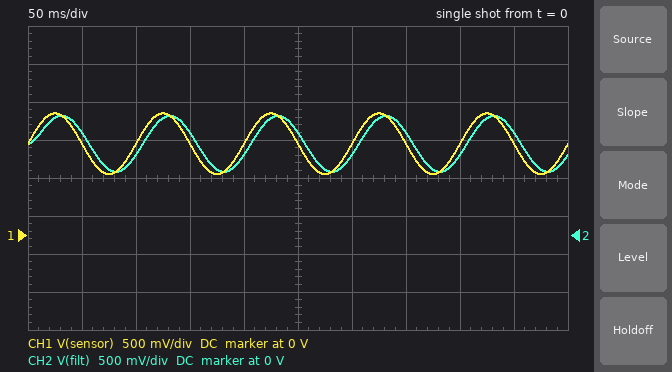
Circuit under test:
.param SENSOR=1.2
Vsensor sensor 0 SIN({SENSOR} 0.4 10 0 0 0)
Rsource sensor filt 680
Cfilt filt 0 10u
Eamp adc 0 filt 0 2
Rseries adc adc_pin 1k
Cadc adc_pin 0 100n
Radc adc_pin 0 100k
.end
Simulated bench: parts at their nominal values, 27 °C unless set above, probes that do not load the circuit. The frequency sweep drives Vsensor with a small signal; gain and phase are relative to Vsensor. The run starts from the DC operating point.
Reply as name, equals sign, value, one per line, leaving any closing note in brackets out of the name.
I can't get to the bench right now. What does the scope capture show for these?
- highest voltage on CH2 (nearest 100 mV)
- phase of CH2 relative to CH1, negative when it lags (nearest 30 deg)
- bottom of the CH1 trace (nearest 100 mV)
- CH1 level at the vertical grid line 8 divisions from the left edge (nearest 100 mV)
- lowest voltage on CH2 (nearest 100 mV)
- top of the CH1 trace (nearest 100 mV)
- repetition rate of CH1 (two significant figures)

highest voltage on CH2 = 1.6 V
phase of CH2 relative to CH1, negative when it lags = -30 deg
bottom of the CH1 trace = 800 mV
CH1 level at the vertical grid line 8 divisions from the left edge = 1.2 V
lowest voltage on CH2 = 800 mV
top of the CH1 trace = 1.6 V
repetition rate of CH1 = 10 Hz
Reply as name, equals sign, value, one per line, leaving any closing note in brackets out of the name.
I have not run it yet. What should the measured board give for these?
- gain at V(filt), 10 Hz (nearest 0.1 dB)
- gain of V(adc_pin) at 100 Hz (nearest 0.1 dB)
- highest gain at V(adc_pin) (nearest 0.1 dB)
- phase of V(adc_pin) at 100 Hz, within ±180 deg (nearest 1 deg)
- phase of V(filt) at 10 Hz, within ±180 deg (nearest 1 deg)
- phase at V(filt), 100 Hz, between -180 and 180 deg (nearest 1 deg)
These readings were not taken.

gain at V(filt), 10 Hz = -0.7 dB
gain of V(adc_pin) at 100 Hz = -6.9 dB
highest gain at V(adc_pin) = 5.9 dB
phase of V(adc_pin) at 100 Hz, within ±180 deg = -80 deg
phase of V(filt) at 10 Hz, within ±180 deg = -23 deg
phase at V(filt), 100 Hz, between -180 and 180 deg = -77 deg
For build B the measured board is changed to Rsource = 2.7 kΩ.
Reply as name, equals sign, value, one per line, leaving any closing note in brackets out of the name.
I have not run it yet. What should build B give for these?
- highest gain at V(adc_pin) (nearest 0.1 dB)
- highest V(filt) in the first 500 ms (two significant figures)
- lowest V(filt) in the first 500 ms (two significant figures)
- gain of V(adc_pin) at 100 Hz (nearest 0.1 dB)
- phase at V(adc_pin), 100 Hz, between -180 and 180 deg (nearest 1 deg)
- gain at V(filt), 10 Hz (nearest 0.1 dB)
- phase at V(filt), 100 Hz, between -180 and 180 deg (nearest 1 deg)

highest gain at V(adc_pin) = 5.9 dB
highest V(filt) in the first 500 ms = 1.4 V
lowest V(filt) in the first 500 ms = 1.0 V
gain of V(adc_pin) at 100 Hz = -18.7 dB
phase at V(adc_pin), 100 Hz, between -180 and 180 deg = -90 deg
gain at V(filt), 10 Hz = -5.9 dB
phase at V(filt), 100 Hz, between -180 and 180 deg = -87 deg
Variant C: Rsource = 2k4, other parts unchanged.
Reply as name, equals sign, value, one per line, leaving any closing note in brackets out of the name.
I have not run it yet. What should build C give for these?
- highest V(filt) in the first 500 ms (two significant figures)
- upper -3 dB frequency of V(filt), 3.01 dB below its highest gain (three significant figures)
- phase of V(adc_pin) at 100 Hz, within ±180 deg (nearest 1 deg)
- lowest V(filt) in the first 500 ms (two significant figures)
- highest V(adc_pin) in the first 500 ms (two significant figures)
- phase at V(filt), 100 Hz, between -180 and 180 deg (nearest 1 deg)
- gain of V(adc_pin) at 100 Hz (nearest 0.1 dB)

highest V(filt) in the first 500 ms = 1.5 V
upper -3 dB frequency of V(filt), 3.01 dB below its highest gain = 6.63 Hz
phase of V(adc_pin) at 100 Hz, within ±180 deg = -90 deg
lowest V(filt) in the first 500 ms = 980 mV
highest V(adc_pin) in the first 500 ms = 2.9 V
phase at V(filt), 100 Hz, between -180 and 180 deg = -86 deg
gain of V(adc_pin) at 100 Hz = -17.7 dB
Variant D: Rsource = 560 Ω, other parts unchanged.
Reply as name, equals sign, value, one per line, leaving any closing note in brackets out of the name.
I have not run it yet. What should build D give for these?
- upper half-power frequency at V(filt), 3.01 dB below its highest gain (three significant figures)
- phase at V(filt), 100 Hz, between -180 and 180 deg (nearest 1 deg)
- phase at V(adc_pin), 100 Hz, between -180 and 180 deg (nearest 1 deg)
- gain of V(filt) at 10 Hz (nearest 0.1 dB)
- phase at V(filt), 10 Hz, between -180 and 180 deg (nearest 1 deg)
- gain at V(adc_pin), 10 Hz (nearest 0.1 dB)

upper half-power frequency at V(filt), 3.01 dB below its highest gain = 28.4 Hz
phase at V(filt), 100 Hz, between -180 and 180 deg = -74 deg
phase at V(adc_pin), 100 Hz, between -180 and 180 deg = -78 deg
gain of V(filt) at 10 Hz = -0.5 dB
phase at V(filt), 10 Hz, between -180 and 180 deg = -19 deg
gain at V(adc_pin), 10 Hz = 5.4 dB
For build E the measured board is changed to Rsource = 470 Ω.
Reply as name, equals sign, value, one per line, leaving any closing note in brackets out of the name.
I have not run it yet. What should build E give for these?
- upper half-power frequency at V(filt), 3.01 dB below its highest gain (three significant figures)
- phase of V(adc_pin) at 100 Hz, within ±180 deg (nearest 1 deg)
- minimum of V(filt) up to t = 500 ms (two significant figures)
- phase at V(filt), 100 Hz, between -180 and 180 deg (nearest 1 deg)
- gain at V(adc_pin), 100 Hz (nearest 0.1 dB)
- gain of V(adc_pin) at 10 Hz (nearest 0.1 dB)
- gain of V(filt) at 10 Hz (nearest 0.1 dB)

upper half-power frequency at V(filt), 3.01 dB below its highest gain = 33.9 Hz
phase of V(adc_pin) at 100 Hz, within ±180 deg = -75 deg
minimum of V(filt) up to t = 500 ms = 820 mV
phase at V(filt), 100 Hz, between -180 and 180 deg = -71 deg
gain at V(adc_pin), 100 Hz = -4.0 dB
gain of V(adc_pin) at 10 Hz = 5.6 dB
gain of V(filt) at 10 Hz = -0.4 dB
